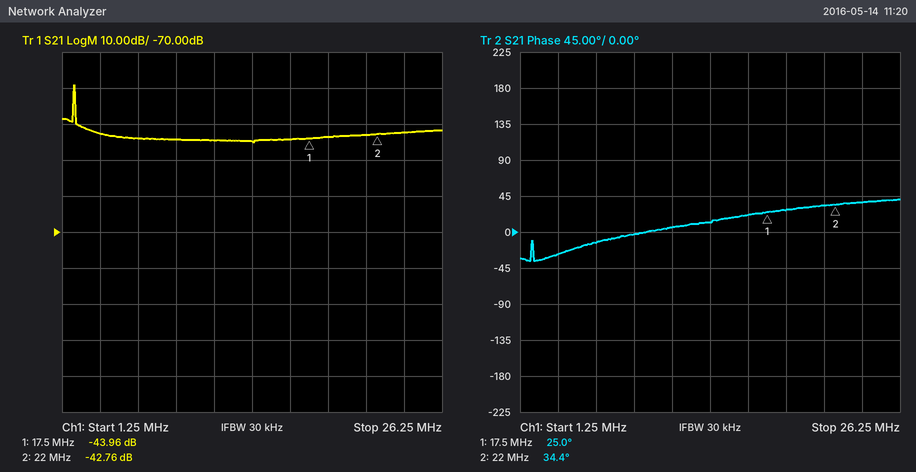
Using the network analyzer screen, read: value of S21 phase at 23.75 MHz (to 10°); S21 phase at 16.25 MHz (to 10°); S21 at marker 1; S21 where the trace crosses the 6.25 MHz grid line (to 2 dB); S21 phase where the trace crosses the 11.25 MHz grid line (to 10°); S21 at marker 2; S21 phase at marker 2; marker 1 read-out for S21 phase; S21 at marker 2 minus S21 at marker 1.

40°
20°
-43.96 dB
-44 dB
10°
-42.76 dB
34.4°
25.0°
1.20 dB
